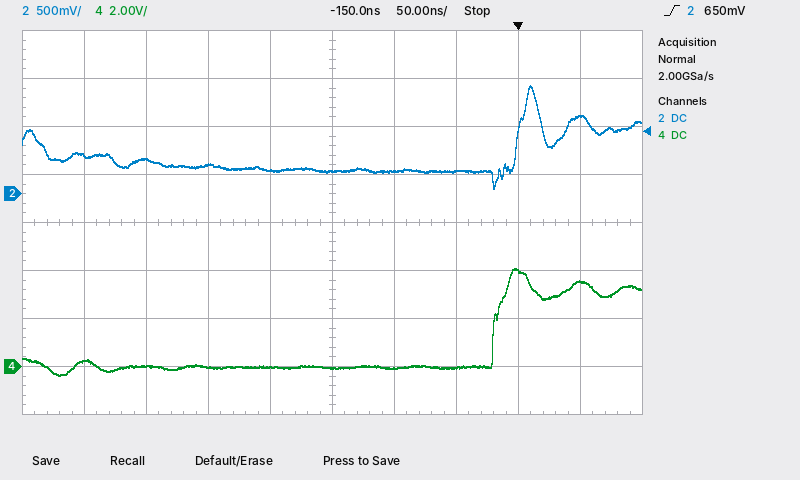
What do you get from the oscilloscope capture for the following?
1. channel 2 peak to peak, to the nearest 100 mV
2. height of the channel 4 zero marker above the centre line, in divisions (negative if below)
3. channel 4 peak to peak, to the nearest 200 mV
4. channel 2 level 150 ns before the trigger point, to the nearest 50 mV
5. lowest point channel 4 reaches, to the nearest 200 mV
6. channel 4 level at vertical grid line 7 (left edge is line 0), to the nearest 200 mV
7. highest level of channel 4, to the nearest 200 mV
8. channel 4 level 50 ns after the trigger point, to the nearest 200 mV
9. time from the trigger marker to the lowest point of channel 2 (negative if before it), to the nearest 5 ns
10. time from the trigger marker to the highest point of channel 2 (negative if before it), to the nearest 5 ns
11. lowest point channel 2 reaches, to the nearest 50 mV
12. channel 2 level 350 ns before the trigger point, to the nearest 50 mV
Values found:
1.10 V
-3.0 div
4.4 V
250 mV
-400 mV
0.0 V
4.0 V
3.6 V
-20 ns
+10 ns
50 mV
400 mV
